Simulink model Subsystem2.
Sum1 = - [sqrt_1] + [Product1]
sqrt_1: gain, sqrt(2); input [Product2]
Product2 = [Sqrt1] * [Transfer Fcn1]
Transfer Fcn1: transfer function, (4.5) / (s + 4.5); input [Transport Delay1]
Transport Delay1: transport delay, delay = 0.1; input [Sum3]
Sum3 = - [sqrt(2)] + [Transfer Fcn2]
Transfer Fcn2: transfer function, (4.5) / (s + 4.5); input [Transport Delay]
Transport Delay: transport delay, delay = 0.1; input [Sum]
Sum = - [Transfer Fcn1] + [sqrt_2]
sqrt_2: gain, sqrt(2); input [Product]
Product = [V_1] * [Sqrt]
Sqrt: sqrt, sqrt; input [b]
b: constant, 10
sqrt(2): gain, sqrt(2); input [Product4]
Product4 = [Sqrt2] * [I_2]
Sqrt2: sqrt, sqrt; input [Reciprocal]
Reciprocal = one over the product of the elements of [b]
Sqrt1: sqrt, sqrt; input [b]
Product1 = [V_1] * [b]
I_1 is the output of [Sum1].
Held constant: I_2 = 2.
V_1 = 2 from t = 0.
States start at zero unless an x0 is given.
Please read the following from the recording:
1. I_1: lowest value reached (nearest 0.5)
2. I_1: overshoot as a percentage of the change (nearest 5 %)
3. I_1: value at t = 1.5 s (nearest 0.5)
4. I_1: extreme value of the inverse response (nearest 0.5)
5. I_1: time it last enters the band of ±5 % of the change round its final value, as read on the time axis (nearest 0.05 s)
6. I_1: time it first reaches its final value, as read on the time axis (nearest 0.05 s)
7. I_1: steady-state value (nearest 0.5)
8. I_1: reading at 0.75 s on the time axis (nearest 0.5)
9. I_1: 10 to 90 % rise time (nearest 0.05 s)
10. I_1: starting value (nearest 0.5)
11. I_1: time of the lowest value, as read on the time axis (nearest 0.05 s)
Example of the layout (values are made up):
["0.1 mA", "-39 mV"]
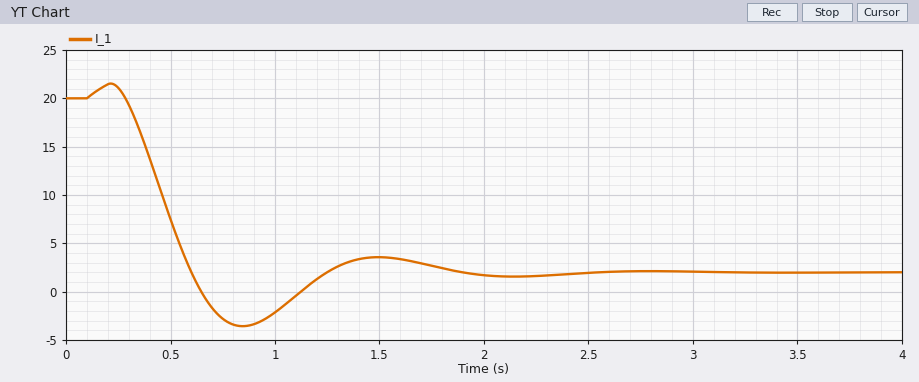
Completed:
["-3.5", "30 %", "3.5", "21.5", "1.70 s", "0.60 s", "2.0", "-3.0", "0.25 s", "20.0", "0.85 s"]
